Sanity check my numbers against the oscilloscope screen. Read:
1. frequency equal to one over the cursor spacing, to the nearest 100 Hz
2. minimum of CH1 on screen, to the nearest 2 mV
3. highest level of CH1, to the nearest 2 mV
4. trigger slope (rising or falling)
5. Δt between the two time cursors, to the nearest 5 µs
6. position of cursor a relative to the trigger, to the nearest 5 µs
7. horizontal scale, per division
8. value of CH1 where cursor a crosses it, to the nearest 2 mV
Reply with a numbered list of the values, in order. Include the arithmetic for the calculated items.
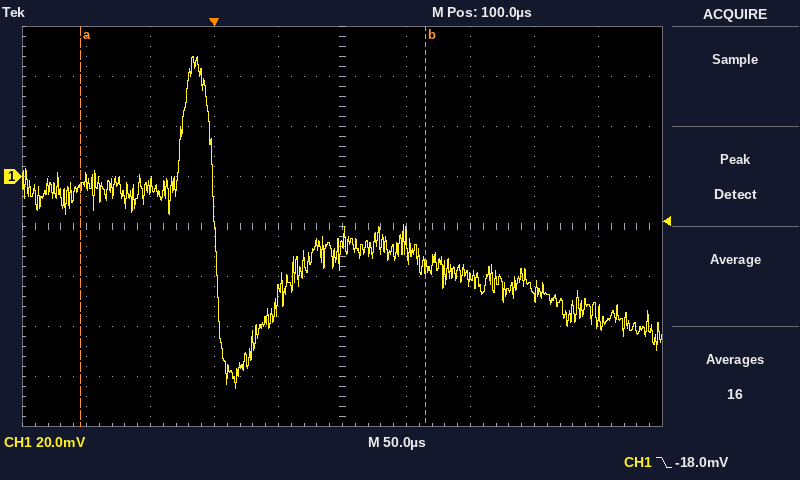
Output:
1. 1 / 270 µs ≈ 3.7 kHz
2. -84 mV
3. 48 mV
4. falling
5. 270 µs
6. -105 µs
7. 50 µs
8. -4 mV
